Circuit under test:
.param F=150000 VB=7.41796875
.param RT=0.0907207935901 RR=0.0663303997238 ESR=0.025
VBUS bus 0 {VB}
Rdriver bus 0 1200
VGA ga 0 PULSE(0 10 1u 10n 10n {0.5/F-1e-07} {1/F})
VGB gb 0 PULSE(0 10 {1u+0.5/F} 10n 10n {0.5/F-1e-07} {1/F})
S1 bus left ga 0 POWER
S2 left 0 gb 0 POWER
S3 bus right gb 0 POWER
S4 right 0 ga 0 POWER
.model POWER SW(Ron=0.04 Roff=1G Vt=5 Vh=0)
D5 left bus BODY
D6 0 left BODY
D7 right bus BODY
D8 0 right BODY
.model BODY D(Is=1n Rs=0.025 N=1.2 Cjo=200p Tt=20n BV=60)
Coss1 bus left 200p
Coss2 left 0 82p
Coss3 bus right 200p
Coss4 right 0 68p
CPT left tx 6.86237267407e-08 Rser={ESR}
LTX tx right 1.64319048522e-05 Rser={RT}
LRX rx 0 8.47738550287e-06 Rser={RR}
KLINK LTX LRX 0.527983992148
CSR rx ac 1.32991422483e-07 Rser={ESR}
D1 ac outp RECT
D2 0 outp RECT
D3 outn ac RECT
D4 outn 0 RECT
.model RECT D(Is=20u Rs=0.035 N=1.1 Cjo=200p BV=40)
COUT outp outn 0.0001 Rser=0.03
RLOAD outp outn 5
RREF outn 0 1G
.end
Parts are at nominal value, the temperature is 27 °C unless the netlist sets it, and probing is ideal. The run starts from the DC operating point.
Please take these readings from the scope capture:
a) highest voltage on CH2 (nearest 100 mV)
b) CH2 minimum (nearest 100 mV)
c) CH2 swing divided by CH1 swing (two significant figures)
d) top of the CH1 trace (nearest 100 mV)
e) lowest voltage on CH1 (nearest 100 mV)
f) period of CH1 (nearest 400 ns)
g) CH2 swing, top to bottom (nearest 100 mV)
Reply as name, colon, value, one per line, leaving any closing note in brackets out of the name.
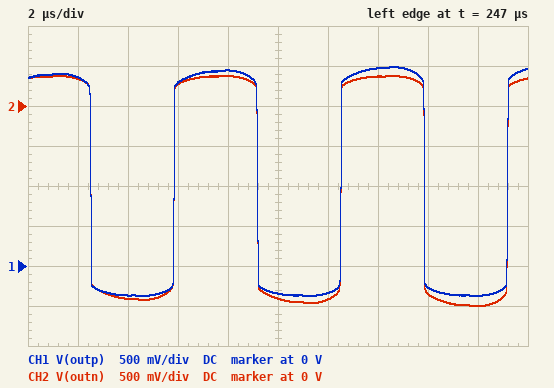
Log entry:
highest voltage on CH2: 400 mV
CH2 minimum: -2.5 V
CH2 swing divided by CH1 swing: 1.0
top of the CH1 trace: 2.5 V
lowest voltage on CH1: -400 mV
period of CH1: 6.8 µs
CH2 swing, top to bottom: 2.9 V
